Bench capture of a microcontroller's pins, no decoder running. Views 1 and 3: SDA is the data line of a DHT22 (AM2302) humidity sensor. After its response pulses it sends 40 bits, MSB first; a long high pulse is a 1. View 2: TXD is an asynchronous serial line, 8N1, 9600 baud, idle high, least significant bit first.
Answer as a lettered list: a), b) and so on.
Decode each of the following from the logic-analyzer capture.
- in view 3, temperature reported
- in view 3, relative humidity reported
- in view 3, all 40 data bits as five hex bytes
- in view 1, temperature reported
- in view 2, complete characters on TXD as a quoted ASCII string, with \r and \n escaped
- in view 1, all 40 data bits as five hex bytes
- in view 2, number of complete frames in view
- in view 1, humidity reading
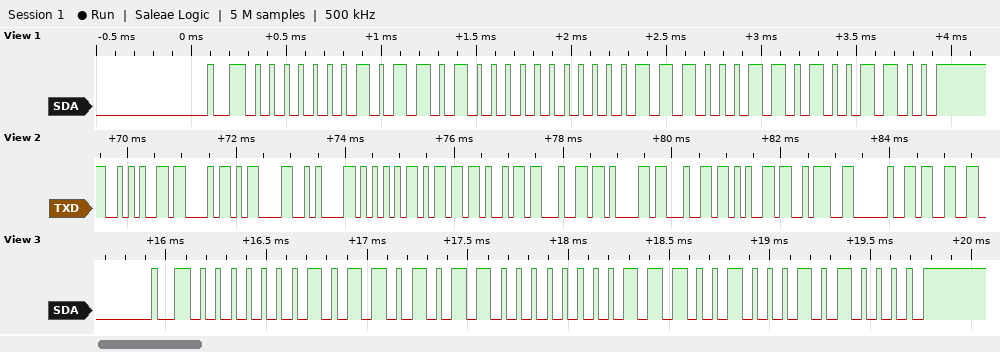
a) 22.8 °C
b) 36.3 %
c) 01 6B 00 E4 50
d) 22.7 °C
e) "*C\r\nUmidade: 3"
f) 01 68 00 E3 4C
g) 14
h) 36.0 %
